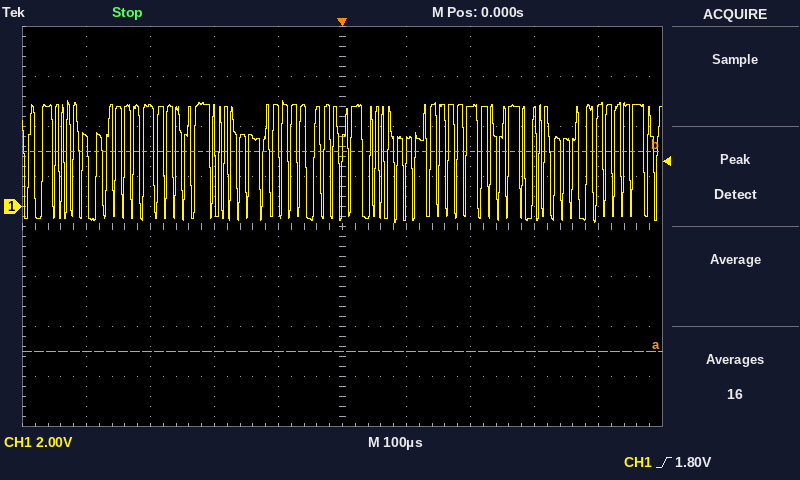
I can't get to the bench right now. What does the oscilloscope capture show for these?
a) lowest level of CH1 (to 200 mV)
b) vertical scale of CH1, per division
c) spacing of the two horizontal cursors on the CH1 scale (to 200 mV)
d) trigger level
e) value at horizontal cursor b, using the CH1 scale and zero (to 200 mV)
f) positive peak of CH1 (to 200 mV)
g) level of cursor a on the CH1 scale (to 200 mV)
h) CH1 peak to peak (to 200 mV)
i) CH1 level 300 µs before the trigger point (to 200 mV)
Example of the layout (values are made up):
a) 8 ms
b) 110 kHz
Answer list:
a) -600 mV
b) 2 V
c) 8.0 V
d) 1.80 V
e) 2.2 V
f) 4.2 V
g) -5.8 V
h) 4.8 V
i) 4.0 V
